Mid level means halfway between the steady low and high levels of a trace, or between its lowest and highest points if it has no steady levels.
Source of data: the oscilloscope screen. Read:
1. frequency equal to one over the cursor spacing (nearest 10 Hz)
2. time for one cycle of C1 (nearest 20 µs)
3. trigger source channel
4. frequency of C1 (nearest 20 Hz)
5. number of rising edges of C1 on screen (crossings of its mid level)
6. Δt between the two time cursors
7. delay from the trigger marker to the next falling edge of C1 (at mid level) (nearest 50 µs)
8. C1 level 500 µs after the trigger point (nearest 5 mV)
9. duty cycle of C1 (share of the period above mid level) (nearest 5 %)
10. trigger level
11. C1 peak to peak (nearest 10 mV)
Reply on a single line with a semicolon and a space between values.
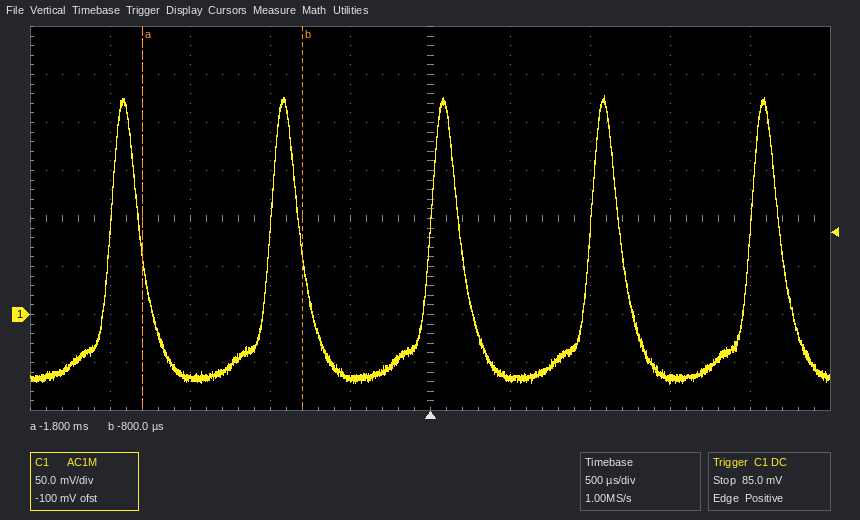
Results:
1.00 kHz; 1.00 ms; C1; 1.00 kHz; 5; 1.00 ms; 200 µs; -65 mV; 20 %; 85.0 mV; 300 mV
